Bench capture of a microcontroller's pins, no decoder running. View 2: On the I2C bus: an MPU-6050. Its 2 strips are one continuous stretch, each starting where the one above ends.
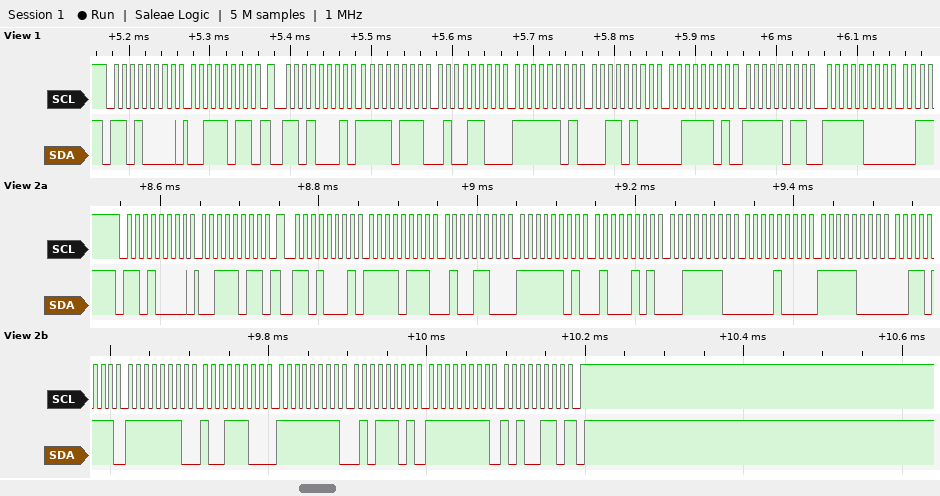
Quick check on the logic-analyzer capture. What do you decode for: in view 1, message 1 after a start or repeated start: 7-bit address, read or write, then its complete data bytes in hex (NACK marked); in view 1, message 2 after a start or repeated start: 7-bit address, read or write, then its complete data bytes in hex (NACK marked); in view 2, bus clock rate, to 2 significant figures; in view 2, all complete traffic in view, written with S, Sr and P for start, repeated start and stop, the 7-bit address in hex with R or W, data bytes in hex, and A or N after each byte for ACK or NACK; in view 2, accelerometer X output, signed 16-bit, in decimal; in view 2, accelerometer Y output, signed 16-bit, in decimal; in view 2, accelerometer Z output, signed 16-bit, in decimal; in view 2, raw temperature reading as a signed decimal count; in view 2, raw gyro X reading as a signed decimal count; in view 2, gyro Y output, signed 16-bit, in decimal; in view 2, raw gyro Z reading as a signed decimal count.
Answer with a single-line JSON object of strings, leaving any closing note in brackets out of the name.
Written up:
{"in view 1, message 1 after a start or repeated start: 7-bit address, read or write, then its complete data bytes in hex": "0x68 write: 3B", "in view 1, message 2 after a start or repeated start: 7-bit address, read or write, then its complete data bytes in hex": "0x68 read: F7 4C FD 34 3D FB F8", "in view 2, bus clock rate, to 2 significant figures": "100 kHz", "in view 2, all complete traffic in view, written with S, Sr and P for start, repeated start and stop, the 7-bit address in hex with R or W, data bytes in hex, and A or N after each byte for ACK or NACK": "S 68W A 3B A Sr 68R A F7 A 4C A FD A 45 A 3E A 08 A F8 A 37 A FE A 9C A FF A 5D A FF A A6 N P", "in view 2, accelerometer X output, signed 16-bit, in decimal": "-2228", "in view 2, accelerometer Y output, signed 16-bit, in decimal": "-699", "in view 2, accelerometer Z output, signed 16-bit, in decimal": "15880", "in view 2, raw temperature reading as a signed decimal count": "-1993", "in view 2, raw gyro X reading as a signed decimal count": "-356", "in view 2, gyro Y output, signed 16-bit, in decimal": "-163", "in view 2, raw gyro Z reading as a signed decimal count": "-90"}
